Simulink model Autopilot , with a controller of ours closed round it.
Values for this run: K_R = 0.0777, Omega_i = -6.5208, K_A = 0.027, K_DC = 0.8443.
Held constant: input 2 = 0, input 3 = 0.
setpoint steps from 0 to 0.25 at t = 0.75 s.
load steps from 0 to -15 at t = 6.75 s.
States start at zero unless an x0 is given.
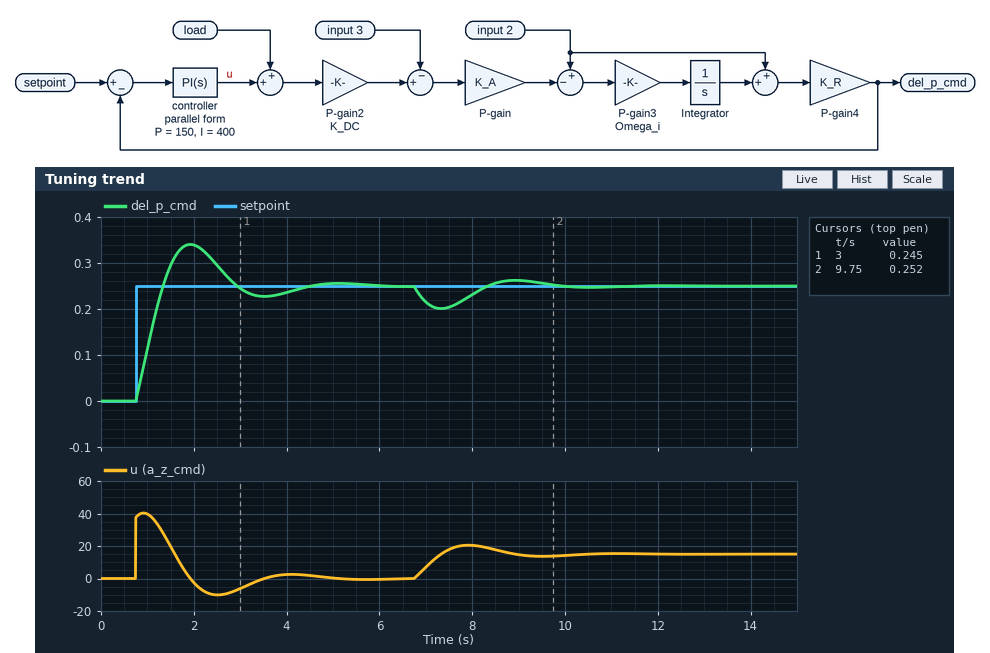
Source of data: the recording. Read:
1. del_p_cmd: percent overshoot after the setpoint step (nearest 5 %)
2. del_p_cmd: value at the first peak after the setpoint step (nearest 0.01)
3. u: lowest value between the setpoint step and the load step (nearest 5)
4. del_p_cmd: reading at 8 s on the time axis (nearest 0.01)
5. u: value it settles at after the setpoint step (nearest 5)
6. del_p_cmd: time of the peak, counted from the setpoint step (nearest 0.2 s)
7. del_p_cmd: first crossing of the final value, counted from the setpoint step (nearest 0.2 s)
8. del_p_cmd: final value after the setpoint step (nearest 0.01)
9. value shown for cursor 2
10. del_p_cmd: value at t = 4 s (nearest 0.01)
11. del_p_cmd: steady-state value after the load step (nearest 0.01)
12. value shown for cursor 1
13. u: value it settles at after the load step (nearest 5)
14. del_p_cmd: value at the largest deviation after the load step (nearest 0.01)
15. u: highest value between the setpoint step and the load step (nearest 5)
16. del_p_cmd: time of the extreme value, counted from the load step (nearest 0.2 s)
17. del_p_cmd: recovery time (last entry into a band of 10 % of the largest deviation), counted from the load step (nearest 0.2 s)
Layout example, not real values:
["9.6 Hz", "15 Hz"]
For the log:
["35 %", "0.34", "-10", "0.23", "0", "1.2 s", "0.6 s", "0.25", "0.252", "0.24", "0.25", "0.245", "15", "0.20", "40", "0.6 s", "2.8 s"]
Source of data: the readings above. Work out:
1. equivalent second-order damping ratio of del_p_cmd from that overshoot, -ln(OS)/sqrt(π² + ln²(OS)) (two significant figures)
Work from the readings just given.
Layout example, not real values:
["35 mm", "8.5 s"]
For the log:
["0.32"]
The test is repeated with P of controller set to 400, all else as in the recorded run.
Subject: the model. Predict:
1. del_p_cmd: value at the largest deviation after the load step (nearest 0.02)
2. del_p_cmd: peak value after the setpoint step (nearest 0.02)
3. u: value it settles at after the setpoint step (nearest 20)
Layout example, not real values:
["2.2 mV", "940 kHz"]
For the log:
["0.22", "0.28", "0"]
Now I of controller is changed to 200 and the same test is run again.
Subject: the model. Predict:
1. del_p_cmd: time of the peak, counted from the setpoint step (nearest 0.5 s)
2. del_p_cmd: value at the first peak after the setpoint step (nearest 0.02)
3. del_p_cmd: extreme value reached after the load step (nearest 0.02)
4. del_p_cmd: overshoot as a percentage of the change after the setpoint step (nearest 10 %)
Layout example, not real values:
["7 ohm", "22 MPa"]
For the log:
["1.5 s", "0.32", "0.20", "30 %"]
